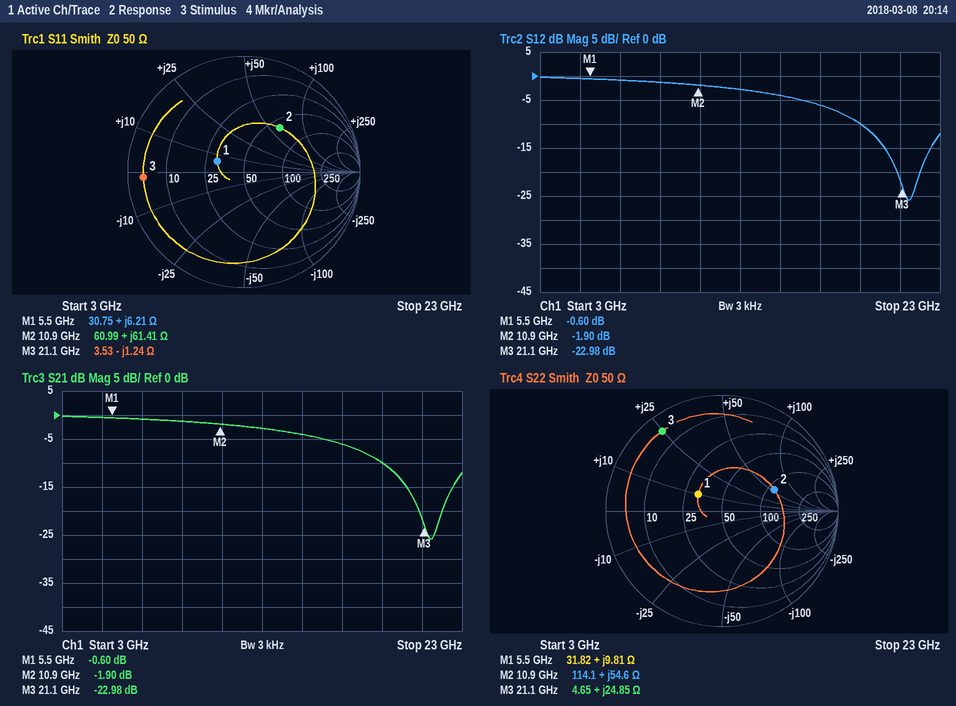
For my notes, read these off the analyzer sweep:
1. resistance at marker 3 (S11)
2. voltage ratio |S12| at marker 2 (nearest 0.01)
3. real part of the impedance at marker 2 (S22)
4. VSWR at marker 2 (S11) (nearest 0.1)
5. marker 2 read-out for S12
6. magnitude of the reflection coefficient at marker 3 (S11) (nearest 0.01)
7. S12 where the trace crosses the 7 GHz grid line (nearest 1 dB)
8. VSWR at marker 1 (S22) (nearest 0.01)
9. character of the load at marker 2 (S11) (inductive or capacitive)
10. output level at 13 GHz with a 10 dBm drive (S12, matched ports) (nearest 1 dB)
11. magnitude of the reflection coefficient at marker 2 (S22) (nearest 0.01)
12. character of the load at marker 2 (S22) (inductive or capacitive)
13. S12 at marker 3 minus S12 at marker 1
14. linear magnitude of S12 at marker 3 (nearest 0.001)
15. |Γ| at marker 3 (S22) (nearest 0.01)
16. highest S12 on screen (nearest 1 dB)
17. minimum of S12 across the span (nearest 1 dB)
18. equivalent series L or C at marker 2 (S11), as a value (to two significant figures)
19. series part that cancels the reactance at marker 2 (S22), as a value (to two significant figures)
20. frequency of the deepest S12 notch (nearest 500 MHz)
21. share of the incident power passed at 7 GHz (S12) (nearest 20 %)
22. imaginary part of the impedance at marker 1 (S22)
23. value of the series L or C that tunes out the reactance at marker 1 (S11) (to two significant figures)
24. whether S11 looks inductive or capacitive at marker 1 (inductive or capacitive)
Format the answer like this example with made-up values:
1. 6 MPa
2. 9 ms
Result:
1. 3.53 Ω
2. 0.80
3. 114.1 Ω
4. 2.9
5. -1.90 dB
6. 0.87
7. -1 dB
8. 1.67
9. inductive
10. 7 dBm
11. 0.49
12. inductive
13. -22.38 dB
14. 0.071
15. 0.86
16. 0 dB
17. -26 dB
18. 900 pH
19. 270 fF
20. 21.5 GHz
21. 80 %
22. +9.81 Ω
23. 4.7 pF
24. inductive
